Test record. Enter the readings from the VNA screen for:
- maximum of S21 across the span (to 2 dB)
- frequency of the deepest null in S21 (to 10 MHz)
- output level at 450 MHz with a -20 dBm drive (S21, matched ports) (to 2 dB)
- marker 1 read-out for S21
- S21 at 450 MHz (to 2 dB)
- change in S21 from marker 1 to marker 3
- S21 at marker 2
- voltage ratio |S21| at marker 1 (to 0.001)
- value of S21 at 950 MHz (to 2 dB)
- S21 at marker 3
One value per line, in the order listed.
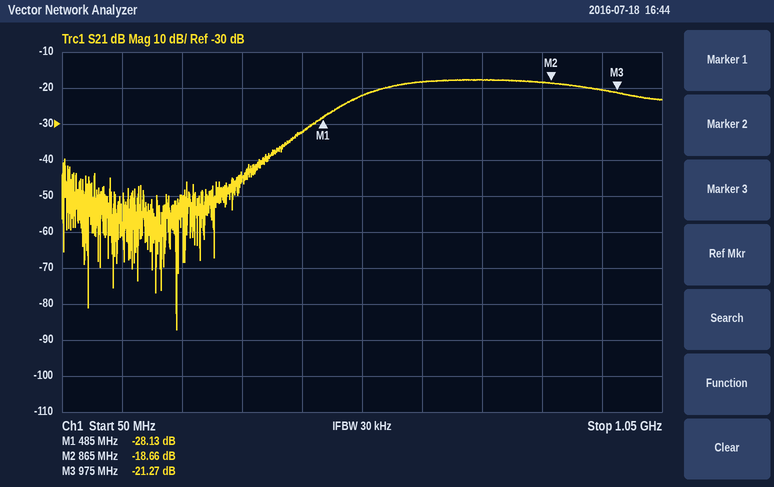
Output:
-18 dB
240 MHz
-52 dBm
-28.13 dB
-32 dB
6.86 dB
-18.66 dB
0.039
-20 dB
-21.27 dB
